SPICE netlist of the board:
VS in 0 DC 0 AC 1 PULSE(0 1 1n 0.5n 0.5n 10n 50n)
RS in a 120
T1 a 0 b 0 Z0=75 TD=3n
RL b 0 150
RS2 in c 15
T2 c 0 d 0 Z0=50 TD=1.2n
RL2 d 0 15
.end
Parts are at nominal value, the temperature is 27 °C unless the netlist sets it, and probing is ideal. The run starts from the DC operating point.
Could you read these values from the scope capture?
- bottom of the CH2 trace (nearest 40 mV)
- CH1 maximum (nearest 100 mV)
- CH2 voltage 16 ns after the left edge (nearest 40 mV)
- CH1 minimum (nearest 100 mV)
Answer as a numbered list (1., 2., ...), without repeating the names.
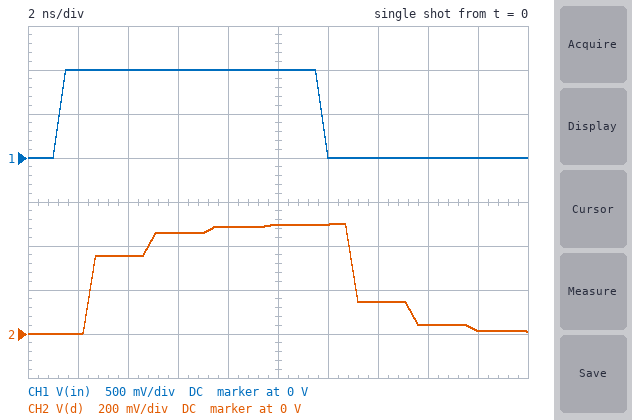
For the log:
1. 0 V
2. 1.0 V
3. 40 mV
4. 0 V
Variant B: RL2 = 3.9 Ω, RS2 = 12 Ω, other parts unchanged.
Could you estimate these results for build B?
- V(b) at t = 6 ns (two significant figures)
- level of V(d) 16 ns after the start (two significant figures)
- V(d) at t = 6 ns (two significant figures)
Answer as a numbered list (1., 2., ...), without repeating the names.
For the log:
1. 510 mV
2. 62 mV
3. 180 mV
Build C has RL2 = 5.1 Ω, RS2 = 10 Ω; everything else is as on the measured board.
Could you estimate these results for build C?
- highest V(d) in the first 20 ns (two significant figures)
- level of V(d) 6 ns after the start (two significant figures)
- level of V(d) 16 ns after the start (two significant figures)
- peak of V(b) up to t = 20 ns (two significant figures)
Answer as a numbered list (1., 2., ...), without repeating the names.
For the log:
1. 320 mV
2. 240 mV
3. 91 mV
4. 550 mV
